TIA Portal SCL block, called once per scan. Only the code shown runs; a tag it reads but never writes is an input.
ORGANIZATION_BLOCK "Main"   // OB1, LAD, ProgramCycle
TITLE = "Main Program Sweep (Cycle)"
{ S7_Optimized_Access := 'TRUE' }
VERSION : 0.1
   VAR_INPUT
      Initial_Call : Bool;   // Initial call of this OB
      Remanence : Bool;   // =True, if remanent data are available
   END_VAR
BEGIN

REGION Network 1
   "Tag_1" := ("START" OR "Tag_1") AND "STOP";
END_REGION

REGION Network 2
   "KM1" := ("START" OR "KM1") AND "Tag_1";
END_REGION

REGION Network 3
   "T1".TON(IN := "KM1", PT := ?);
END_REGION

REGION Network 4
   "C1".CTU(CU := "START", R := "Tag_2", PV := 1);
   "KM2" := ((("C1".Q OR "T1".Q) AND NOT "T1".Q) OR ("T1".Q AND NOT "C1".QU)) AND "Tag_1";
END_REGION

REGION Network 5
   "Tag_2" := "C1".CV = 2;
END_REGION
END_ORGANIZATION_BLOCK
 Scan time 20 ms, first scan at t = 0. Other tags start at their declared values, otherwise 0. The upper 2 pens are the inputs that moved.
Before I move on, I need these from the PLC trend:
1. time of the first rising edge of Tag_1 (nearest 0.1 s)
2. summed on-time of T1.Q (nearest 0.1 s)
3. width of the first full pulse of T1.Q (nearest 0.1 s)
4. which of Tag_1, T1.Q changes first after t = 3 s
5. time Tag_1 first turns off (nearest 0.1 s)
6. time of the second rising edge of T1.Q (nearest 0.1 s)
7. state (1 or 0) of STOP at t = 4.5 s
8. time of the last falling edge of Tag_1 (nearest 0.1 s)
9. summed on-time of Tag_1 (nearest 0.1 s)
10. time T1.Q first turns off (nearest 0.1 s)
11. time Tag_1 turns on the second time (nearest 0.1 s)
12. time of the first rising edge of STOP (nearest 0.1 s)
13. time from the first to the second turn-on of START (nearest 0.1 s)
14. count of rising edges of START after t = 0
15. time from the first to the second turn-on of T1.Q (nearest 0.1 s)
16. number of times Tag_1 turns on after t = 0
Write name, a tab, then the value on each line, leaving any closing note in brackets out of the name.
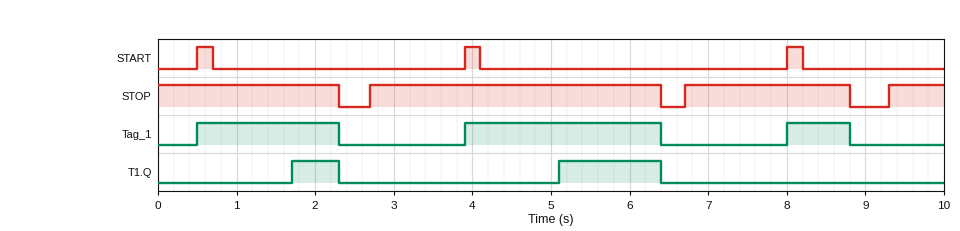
time of the first rising edge of Tag_1	0.5 s
summed on-time of T1.Q	1.9 s
width of the first full pulse of T1.Q	0.6 s
which of Tag_1, T1.Q changes first after t = 3 s	Tag_1
time Tag_1 first turns off	2.3 s
time of the second rising edge of T1.Q	5.1 s
state (1 or 0) of STOP at t = 4.5 s	1
time of the last falling edge of Tag_1	8.8 s
summed on-time of Tag_1	5.1 s
time T1.Q first turns off	2.3 s
time Tag_1 turns on the second time	3.9 s
time of the first rising edge of STOP	2.7 s
time from the first to the second turn-on of START	3.4 s
count of rising edges of START after t = 0	3
time from the first to the second turn-on of T1.Q	3.4 s
number of times Tag_1 turns on after t = 0	3
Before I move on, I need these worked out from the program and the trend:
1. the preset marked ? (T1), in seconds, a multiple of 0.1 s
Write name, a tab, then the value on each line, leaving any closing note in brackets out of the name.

the preset marked ? (T1), in seconds, a multiple of 0.1 s	1.2 s
